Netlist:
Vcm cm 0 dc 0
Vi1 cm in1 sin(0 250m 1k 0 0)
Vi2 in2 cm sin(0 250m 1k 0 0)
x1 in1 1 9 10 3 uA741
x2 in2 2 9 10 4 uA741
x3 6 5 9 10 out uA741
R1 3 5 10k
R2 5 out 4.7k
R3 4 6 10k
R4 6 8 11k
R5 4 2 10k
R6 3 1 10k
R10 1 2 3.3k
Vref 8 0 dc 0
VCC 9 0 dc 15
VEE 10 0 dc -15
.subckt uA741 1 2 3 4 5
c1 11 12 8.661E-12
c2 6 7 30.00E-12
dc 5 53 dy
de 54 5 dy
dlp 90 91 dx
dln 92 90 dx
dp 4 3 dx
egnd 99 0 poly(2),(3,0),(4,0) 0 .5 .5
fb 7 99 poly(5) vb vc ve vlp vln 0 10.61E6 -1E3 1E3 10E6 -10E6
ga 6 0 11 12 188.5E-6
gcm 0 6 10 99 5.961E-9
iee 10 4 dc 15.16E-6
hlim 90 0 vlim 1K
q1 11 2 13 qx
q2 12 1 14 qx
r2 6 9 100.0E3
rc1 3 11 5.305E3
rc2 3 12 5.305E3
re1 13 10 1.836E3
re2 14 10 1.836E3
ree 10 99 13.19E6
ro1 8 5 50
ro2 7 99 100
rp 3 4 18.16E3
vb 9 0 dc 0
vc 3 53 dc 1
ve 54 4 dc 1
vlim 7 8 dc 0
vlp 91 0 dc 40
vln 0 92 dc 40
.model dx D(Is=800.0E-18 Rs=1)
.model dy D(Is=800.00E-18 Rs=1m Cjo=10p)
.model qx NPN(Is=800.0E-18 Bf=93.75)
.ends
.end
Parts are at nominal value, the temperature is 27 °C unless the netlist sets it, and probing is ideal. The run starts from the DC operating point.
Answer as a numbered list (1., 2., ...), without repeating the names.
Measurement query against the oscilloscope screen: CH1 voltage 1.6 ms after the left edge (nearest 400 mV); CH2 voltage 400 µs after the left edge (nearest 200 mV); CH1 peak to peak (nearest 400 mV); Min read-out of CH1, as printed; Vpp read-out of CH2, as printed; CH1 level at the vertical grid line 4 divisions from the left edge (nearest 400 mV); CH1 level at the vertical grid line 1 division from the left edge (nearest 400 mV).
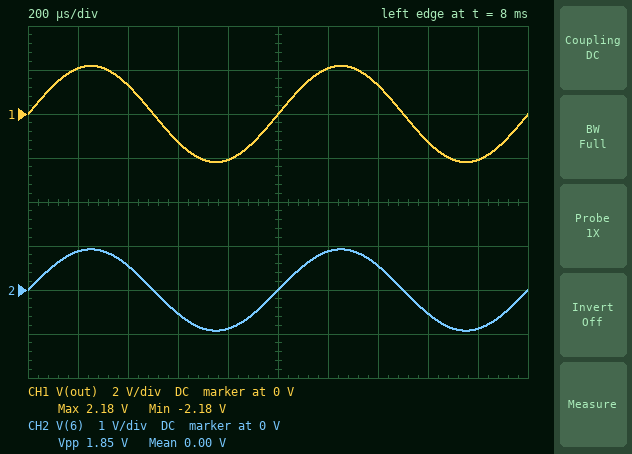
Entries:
1. -1.2 V
2. 600 mV
3. 4.4 V
4. -2.18 V
5. 1.85 V
6. -2.0 V
7. 2.0 V
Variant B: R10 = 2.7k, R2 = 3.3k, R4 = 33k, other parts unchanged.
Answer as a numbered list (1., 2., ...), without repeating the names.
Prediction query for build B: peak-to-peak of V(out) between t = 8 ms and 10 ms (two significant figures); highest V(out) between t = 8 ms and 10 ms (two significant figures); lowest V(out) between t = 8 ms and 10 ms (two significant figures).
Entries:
1. 5.7 V
2. 2.8 V
3. -2.8 V
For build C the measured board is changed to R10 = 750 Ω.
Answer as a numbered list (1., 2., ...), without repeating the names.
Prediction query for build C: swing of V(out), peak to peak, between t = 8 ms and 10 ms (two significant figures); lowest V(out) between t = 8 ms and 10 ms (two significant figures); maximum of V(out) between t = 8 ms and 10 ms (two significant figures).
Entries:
1. 17 V
2. -8.6 V
3. 8.6 V
